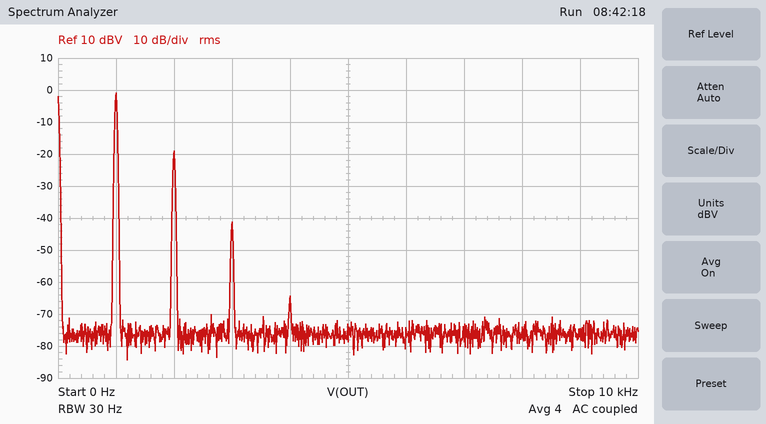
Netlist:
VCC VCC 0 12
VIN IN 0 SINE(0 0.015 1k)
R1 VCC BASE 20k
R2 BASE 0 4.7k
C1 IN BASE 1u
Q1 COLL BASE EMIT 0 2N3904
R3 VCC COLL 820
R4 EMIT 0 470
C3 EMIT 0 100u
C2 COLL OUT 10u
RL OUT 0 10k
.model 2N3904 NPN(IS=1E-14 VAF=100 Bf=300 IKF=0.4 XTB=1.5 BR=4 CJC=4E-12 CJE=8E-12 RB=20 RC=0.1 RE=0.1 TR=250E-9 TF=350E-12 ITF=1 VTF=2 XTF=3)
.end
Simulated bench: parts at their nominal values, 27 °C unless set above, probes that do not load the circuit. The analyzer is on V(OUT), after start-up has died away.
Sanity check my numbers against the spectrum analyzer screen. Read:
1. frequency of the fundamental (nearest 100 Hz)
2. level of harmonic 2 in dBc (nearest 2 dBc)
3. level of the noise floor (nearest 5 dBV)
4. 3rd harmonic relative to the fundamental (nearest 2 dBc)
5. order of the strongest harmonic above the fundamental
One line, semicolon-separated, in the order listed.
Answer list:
1.0 kHz; -18 dBc; -75 dBV; -40 dBc; 2
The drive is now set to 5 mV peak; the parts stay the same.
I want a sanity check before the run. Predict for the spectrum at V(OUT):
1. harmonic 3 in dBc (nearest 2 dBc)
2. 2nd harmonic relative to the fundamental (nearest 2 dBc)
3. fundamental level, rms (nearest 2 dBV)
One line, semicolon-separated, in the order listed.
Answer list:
-60 dBc; -28 dBc; -10 dBV
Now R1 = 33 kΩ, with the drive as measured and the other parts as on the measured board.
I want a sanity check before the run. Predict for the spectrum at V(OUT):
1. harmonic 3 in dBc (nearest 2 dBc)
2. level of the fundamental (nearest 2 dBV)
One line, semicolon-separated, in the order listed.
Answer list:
-38 dBc; -6 dBV
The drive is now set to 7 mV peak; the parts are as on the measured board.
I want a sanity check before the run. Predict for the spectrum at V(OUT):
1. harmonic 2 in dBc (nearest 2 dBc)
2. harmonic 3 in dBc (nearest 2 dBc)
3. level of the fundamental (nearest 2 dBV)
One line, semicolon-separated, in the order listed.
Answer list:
-24 dBc; -54 dBc; -8 dBV
